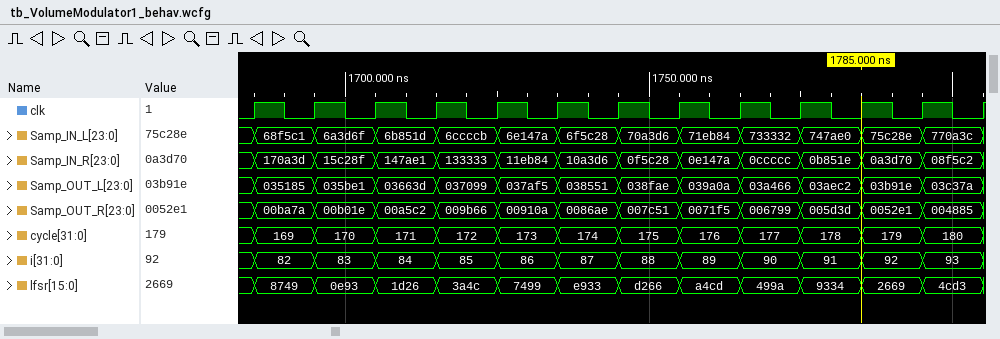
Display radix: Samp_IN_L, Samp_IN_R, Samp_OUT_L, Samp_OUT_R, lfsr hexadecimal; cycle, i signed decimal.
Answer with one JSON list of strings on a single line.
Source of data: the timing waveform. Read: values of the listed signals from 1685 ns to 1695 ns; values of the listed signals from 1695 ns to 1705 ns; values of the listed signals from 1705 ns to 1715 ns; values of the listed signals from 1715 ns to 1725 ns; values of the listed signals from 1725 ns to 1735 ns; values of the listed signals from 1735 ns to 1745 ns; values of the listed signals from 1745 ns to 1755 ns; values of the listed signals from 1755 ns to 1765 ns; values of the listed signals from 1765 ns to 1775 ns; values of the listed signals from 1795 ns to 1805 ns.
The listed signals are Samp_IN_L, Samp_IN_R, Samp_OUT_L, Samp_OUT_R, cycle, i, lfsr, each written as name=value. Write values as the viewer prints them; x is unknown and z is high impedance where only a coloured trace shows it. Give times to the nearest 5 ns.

["Samp_IN_L=68f5c1, Samp_IN_R=170a3d, Samp_OUT_L=035185, Samp_OUT_R=00ba7a, cycle=169, i=82, lfsr=8749", "Samp_IN_L=6a3d6f, Samp_IN_R=15c28f, Samp_OUT_L=035be1, Samp_OUT_R=00b01e, cycle=170, i=83, lfsr=0e93", "Samp_IN_L=6b851d, Samp_IN_R=147ae1, Samp_OUT_L=03663d, Samp_OUT_R=00a5c2, cycle=171, i=84, lfsr=1d26", "Samp_IN_L=6ccccb, Samp_IN_R=133333, Samp_OUT_L=037099, Samp_OUT_R=009b66, cycle=172, i=85, lfsr=3a4c", "Samp_IN_L=6e147a, Samp_IN_R=11eb84, Samp_OUT_L=037af5, Samp_OUT_R=00910a, cycle=173, i=86, lfsr=7499", "Samp_IN_L=6f5c28, Samp_IN_R=10a3d6, Samp_OUT_L=038551, Samp_OUT_R=0086ae, cycle=174, i=87, lfsr=e933", "Samp_IN_L=70a3d6, Samp_IN_R=0f5c28, Samp_OUT_L=038fae, Samp_OUT_R=007c51, cycle=175, i=88, lfsr=d266", "Samp_IN_L=71eb84, Samp_IN_R=0e147a, Samp_OUT_L=039a0a, Samp_OUT_R=0071f5, cycle=176, i=89, lfsr=a4cd", "Samp_IN_L=733332, Samp_IN_R=0ccccc, Samp_OUT_L=03a466, Samp_OUT_R=006799, cycle=177, i=90, lfsr=499a", "Samp_IN_L=770a3c, Samp_IN_R=08f5c2, Samp_OUT_L=03c37a, Samp_OUT_R=004885, cycle=180, i=93, lfsr=4cd3"]
